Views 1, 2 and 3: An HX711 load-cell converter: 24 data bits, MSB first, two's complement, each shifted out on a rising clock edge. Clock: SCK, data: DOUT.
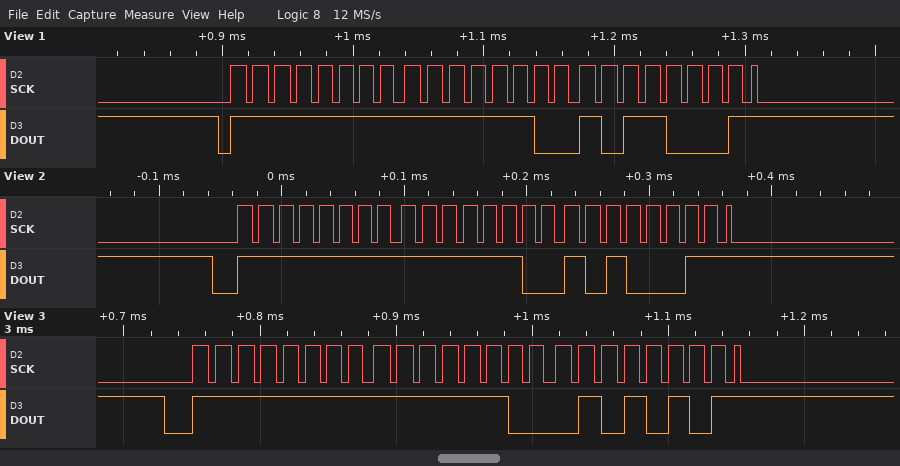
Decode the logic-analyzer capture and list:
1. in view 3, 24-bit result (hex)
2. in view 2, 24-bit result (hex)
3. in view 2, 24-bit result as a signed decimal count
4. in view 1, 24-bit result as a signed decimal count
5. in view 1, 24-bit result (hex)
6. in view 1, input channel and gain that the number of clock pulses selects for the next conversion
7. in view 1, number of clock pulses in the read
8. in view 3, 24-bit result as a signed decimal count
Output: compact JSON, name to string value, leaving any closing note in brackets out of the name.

{"in view 3, 24-bit result": "0xFFFC55", "in view 2, 24-bit result": "0xFFFCA3", "in view 2, 24-bit result as a signed decimal count": "-861", "in view 1, 24-bit result as a signed decimal count": "-847", "in view 1, 24-bit result": "0xFFFCB1", "in view 1, input channel and gain that the number of clock pulses selects for the next conversion": "channel A, gain 128", "in view 1, number of clock pulses in the read": "25", "in view 3, 24-bit result as a signed decimal count": "-939"}
